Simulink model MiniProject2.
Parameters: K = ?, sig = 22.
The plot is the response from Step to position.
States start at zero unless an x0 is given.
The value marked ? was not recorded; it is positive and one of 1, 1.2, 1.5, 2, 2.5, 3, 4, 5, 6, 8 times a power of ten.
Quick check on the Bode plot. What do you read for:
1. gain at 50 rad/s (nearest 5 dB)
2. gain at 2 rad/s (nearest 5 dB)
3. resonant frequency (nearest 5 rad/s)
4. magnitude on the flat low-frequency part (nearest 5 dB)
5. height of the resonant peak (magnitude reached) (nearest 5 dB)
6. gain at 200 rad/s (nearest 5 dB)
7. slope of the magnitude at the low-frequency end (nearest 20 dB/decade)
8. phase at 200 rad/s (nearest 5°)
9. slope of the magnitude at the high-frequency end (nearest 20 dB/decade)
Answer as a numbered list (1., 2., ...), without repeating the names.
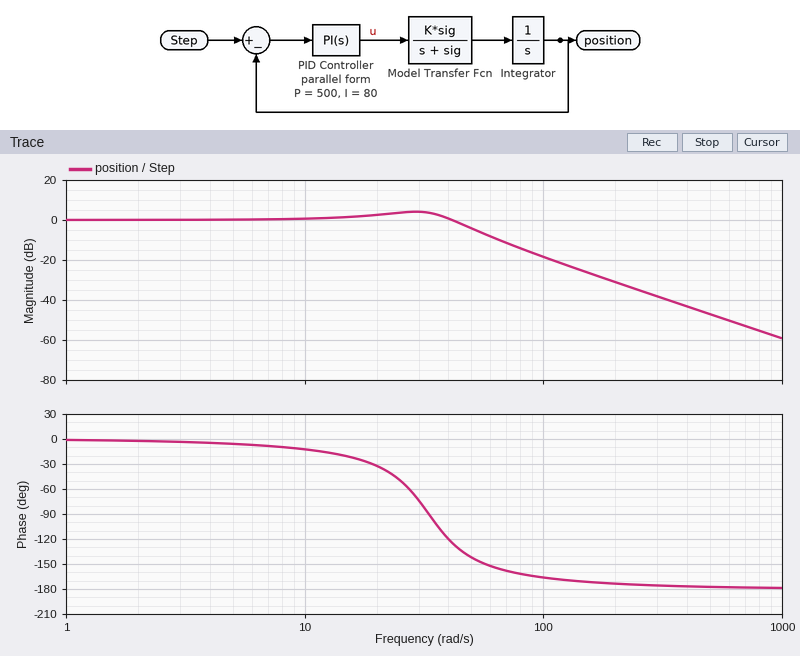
1. -5 dB
2. 0 dB
3. 30 rad/s
4. 0 dB
5. 5 dB
6. -30 dB
7. 0 dB/decade
8. -175°
9. -40 dB/decade
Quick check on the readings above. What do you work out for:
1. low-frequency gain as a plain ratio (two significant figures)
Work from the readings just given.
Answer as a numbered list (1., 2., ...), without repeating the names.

1. 1.0
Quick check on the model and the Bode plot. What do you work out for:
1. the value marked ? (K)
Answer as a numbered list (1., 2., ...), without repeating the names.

1. 0.1
